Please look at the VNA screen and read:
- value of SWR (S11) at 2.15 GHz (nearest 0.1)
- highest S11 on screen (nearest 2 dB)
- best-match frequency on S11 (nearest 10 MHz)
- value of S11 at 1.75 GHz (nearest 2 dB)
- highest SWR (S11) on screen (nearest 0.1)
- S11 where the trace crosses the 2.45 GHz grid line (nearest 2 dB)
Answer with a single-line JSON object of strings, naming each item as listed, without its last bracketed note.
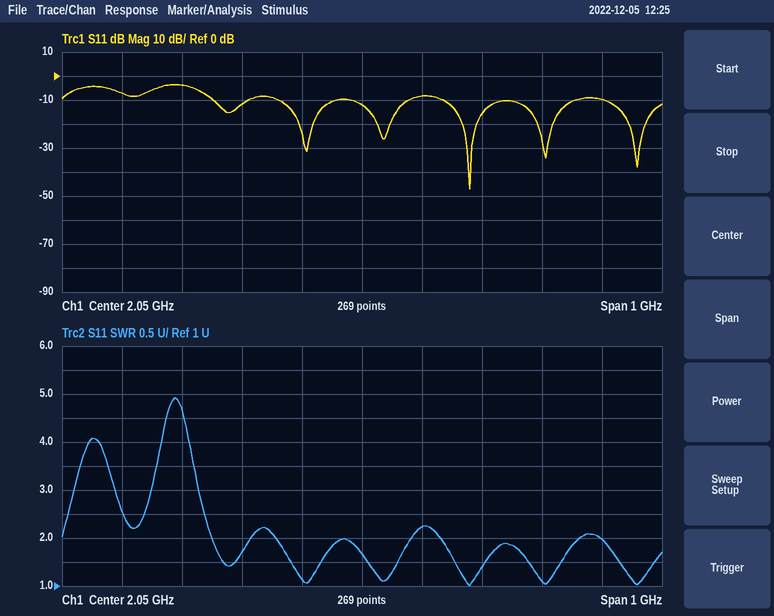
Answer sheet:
{"value of SWR (S11) at 2.15 GHz": "2.2", "highest S11 on screen": "-4 dB", "best-match frequency on S11": "2.23 GHz", "value of S11 at 1.75 GHz": "-4 dB", "highest SWR (S11) on screen": "4.9", "S11 where the trace crosses the 2.45 GHz grid line": "-10 dB"}
